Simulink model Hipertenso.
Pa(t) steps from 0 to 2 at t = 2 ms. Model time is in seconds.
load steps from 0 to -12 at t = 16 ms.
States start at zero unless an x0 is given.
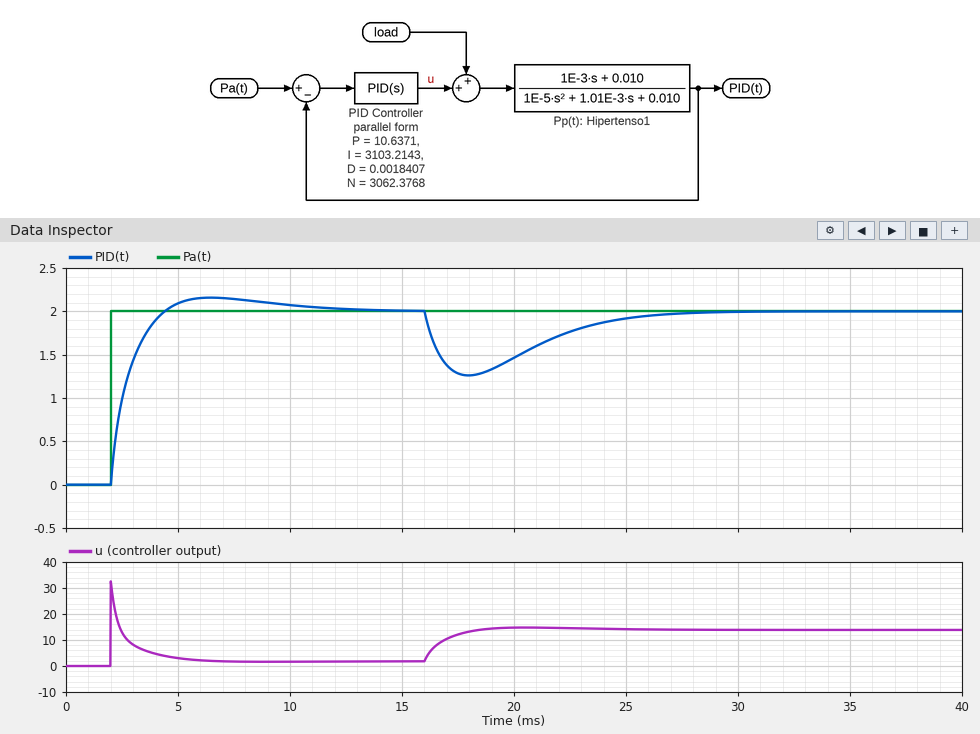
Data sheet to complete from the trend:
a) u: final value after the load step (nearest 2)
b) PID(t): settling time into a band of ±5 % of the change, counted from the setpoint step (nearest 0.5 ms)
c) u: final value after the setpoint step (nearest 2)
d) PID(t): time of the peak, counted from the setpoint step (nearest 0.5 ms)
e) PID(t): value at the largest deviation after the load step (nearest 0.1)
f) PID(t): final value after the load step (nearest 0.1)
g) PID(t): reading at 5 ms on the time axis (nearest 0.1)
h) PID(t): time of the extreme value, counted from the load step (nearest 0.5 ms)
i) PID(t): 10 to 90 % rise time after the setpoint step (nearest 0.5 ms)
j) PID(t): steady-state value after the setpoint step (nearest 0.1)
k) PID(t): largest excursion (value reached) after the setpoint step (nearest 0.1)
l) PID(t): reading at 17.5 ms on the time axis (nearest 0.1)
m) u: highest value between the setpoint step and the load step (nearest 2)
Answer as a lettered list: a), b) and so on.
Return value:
a) 14
b) 7.0 ms
c) 2
d) 4.5 ms
e) 1.3
f) 2.0
g) 2.1
h) 2.0 ms
i) 1.5 ms
j) 2.0
k) 2.2
l) 1.3
m) 32
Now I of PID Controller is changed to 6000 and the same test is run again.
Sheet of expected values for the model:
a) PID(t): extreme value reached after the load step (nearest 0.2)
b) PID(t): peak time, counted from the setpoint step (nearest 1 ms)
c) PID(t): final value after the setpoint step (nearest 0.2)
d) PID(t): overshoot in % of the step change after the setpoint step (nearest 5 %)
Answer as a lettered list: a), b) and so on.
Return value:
a) 1.4
b) 3 ms
c) 2.0
d) 15 %
